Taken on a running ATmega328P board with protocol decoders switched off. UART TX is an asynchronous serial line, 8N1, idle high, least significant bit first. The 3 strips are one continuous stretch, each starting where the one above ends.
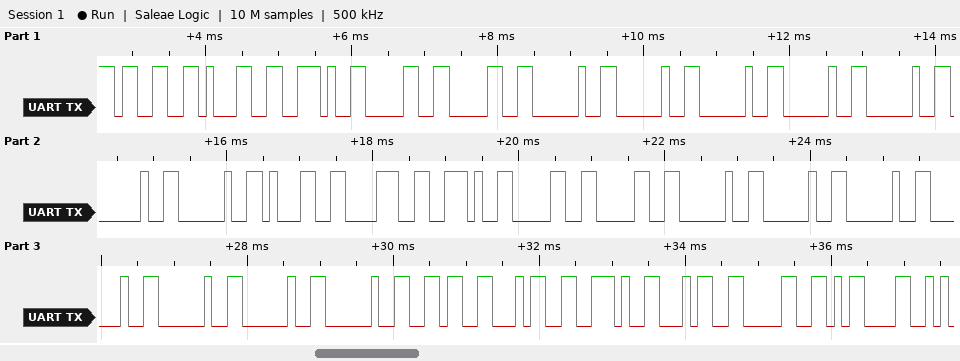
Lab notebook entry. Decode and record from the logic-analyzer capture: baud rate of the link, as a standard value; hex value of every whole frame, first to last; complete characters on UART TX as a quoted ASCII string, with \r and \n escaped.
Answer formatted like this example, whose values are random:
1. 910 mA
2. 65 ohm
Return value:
1. 9600 baud
2. 33 31 2E 30 30 20 20 20 20 20 20 20 31 38 2E 30 30 20 20 20 20 20 20 20 36 34 2E 34 30 0D
3. "31.00       18.00       64.40\r"
